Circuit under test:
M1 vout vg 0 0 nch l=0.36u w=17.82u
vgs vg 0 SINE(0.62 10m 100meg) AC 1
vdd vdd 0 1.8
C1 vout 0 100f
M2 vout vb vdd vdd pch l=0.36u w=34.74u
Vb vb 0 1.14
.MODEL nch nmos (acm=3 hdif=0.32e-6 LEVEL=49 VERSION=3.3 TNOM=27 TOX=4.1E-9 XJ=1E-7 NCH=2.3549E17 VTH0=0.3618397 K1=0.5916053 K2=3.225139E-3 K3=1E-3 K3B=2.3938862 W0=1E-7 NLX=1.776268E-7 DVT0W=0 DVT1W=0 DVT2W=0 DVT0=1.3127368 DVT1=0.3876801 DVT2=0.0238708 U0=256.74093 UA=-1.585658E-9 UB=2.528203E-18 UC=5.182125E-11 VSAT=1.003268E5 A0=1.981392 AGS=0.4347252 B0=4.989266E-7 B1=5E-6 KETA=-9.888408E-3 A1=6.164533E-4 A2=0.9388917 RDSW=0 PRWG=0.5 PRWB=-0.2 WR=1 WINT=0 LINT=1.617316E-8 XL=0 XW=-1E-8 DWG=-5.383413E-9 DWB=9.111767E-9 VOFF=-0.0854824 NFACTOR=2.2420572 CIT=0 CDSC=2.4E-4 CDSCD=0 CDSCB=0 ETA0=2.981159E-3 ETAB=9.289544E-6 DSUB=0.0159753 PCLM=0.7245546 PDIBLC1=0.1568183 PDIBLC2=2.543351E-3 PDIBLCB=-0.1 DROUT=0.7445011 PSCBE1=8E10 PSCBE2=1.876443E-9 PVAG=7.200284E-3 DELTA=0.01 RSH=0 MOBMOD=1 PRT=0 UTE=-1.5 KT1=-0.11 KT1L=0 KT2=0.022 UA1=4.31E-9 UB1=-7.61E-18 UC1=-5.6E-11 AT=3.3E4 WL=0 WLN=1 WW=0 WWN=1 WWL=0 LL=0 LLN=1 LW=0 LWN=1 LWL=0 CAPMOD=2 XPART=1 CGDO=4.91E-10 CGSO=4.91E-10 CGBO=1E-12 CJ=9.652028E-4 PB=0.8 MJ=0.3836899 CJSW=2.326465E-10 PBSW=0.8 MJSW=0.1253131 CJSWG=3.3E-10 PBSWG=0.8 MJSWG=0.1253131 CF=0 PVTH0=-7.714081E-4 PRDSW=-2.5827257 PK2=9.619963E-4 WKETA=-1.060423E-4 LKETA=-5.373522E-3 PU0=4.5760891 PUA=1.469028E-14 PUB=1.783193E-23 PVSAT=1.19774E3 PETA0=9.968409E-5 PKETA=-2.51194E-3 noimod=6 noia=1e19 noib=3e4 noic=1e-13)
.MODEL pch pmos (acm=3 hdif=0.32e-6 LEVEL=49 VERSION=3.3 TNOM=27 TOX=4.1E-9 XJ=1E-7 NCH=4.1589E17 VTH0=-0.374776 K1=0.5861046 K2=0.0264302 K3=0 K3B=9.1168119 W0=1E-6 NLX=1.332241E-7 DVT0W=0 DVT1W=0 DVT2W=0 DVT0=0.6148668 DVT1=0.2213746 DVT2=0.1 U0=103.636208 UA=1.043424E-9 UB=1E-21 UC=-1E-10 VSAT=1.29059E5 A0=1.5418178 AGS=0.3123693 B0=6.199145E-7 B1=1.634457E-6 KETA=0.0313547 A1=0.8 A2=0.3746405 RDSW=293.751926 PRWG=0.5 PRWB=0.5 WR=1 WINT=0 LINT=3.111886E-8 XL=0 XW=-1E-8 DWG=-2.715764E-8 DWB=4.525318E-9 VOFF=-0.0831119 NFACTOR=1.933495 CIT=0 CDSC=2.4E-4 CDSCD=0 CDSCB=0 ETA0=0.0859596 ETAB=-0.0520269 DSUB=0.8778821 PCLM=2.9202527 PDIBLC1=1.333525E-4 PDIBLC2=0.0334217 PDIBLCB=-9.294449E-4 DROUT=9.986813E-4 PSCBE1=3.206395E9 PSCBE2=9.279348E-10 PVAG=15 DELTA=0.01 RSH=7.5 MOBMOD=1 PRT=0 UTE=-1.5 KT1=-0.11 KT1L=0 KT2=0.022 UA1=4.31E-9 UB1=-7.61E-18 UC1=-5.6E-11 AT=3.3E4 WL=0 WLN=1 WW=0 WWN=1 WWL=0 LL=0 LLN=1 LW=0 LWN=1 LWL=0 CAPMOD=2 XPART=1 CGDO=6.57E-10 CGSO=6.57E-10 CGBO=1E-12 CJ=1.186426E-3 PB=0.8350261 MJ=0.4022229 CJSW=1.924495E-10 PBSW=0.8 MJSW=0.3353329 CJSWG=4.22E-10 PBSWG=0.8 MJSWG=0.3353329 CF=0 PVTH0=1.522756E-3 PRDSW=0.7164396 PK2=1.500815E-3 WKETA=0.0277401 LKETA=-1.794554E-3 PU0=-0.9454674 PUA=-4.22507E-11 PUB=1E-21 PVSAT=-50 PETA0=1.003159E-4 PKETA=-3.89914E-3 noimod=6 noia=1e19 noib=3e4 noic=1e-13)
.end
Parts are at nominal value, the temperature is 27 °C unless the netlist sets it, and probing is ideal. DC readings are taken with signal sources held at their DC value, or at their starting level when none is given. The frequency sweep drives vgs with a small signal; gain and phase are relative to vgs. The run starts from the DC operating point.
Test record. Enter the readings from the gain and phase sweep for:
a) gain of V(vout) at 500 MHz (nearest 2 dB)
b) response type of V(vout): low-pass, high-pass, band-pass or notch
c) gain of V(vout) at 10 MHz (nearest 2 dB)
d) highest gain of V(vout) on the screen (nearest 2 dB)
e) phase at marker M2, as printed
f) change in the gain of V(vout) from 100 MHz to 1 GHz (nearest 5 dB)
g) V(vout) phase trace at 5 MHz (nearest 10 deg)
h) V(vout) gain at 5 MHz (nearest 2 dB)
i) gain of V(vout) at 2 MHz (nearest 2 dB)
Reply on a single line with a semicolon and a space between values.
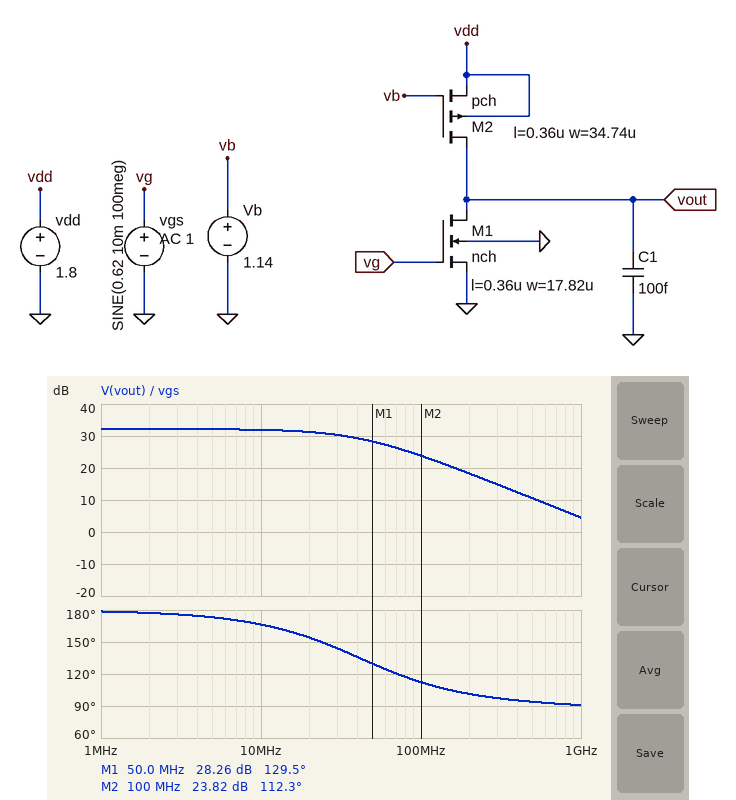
10 dB; low-pass; 32 dB; 32 dB; 112.3 deg; -20 dB; 170 deg; 32 dB; 32 dB
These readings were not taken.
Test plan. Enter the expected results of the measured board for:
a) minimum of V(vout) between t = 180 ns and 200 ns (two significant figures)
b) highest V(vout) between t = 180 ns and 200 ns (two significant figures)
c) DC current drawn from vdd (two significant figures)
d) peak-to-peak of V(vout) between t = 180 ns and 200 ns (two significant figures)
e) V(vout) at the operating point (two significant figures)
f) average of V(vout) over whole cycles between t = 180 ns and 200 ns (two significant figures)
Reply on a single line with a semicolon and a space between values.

910 mV; 1.2 V; 160 µA; 310 mV; 1.1 V; 1.1 V
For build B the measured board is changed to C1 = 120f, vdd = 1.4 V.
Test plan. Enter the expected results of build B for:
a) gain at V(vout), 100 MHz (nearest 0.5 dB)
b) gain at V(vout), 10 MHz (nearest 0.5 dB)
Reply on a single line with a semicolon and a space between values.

-39.5 dB; -59.0 dB
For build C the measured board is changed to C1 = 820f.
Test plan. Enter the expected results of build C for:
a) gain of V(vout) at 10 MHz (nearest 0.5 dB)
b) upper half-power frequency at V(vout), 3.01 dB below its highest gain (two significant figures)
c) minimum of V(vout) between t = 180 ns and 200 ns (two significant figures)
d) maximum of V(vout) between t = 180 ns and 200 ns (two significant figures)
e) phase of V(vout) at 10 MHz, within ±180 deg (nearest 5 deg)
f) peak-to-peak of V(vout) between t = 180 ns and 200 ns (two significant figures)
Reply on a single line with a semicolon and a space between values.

28.5 dB; 8.5 MHz; 1.0 V; 1.1 V; 130 deg; 69 mV
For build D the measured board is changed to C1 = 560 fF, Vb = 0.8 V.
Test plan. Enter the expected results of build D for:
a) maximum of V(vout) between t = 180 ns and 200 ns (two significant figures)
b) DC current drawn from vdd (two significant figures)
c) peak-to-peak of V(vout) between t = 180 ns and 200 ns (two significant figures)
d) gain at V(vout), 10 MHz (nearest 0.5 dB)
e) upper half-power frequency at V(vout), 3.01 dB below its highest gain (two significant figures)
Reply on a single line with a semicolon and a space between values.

1.8 V; 180 µA; 12 mV; -4.5 dB; 710 MHz
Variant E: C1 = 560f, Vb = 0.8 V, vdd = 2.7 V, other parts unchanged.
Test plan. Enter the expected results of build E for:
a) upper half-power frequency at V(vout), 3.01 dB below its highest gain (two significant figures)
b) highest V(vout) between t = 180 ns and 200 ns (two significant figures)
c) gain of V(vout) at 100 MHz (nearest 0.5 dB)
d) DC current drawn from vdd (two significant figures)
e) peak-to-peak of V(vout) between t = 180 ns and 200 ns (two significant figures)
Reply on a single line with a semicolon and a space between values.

1.6 GHz; 2.7 V; -11.0 dB; 200 µA; 5.6 mV
